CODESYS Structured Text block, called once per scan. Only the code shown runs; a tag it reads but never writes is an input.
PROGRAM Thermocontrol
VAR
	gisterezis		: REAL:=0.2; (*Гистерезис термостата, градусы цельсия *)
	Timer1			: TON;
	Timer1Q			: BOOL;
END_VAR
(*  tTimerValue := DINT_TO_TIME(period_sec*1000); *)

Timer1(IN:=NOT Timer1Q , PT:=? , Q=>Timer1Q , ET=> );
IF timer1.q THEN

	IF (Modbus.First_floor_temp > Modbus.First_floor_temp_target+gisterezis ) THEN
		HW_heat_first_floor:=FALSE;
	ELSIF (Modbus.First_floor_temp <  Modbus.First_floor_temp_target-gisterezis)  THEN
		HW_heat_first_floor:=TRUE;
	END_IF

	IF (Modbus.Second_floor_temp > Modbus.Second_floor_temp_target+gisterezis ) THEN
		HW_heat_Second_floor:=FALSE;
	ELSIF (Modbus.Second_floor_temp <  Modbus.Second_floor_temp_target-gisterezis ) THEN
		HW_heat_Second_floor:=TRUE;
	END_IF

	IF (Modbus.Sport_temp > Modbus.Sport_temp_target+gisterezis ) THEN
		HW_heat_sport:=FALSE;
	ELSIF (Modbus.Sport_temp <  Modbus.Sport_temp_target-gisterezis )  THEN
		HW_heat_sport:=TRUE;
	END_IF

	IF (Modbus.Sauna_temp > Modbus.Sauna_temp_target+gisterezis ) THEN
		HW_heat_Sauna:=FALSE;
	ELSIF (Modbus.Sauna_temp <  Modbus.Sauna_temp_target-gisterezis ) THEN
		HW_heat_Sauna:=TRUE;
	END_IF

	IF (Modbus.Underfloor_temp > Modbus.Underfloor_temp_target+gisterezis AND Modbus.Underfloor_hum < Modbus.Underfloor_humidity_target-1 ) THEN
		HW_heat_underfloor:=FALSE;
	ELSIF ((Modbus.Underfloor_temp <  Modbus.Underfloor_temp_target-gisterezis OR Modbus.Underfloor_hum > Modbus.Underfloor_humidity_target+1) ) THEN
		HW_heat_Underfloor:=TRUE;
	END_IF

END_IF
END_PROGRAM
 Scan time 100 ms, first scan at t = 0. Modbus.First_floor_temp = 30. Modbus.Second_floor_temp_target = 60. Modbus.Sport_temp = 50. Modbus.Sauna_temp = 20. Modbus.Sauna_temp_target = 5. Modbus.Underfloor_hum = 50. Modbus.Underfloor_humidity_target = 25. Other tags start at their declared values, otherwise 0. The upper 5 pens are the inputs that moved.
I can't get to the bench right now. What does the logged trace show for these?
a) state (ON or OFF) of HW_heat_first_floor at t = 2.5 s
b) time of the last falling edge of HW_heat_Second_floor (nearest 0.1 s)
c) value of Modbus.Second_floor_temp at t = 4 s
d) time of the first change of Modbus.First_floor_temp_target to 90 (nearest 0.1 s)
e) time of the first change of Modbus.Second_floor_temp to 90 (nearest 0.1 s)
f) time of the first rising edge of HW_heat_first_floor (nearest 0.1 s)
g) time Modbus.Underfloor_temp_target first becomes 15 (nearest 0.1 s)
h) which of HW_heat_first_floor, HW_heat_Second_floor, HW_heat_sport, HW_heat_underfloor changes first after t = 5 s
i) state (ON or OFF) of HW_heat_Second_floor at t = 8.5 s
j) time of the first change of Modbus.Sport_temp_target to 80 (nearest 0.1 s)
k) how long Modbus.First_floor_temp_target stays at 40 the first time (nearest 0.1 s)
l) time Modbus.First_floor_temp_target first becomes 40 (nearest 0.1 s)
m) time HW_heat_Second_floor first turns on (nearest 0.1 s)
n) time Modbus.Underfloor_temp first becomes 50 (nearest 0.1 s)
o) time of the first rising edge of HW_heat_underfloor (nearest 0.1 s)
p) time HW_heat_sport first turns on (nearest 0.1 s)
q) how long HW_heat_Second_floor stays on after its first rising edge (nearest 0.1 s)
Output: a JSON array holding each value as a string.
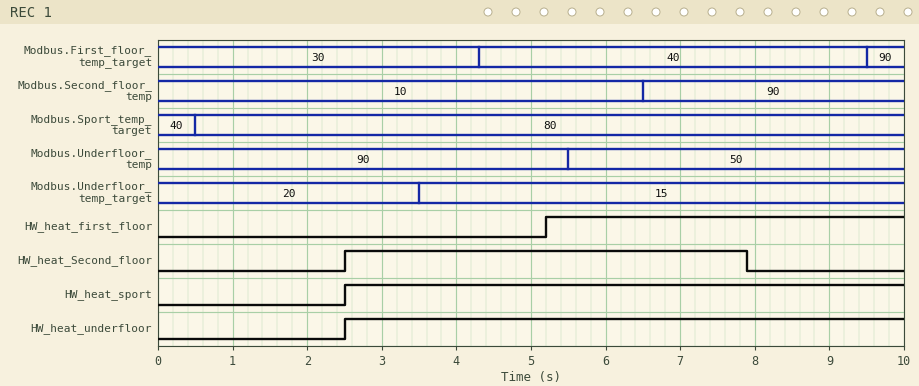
["OFF", "7.9 s", "10", "9.5 s", "6.5 s", "5.2 s", "3.5 s", "HW_heat_first_floor", "OFF", "0.5 s", "5.2 s", "4.3 s", "2.5 s", "5.5 s", "2.5 s", "2.5 s", "5.4 s"]
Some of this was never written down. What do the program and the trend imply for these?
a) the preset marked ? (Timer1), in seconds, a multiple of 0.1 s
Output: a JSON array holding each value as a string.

["2.5 s"]
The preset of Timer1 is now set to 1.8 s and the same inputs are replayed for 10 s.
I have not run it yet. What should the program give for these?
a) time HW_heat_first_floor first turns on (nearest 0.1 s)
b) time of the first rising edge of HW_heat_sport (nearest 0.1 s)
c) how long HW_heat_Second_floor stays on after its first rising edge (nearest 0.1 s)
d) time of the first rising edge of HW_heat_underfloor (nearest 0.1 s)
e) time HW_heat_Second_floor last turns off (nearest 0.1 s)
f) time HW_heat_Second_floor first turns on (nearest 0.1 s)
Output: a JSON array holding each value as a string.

["5.8 s", "1.8 s", "6.0 s", "1.8 s", "7.8 s", "1.8 s"]
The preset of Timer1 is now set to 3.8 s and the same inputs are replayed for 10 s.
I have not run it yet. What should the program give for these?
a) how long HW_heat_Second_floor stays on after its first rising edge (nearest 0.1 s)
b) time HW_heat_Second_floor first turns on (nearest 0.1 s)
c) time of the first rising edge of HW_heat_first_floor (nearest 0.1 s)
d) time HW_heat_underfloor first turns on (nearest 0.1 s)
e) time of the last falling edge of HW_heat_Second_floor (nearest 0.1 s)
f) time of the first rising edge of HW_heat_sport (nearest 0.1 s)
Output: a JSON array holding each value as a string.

["4.0 s", "3.8 s", "7.8 s", "3.8 s", "7.8 s", "3.8 s"]
